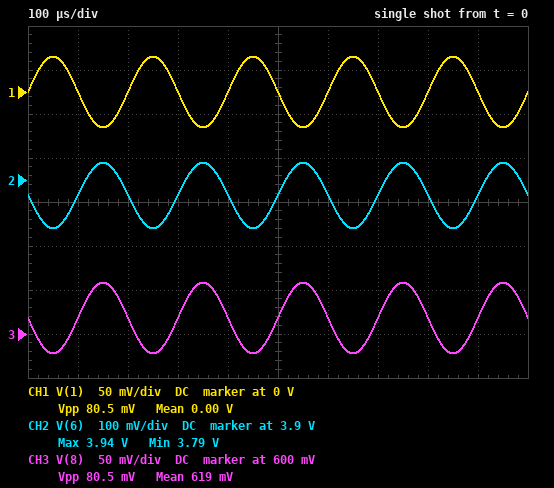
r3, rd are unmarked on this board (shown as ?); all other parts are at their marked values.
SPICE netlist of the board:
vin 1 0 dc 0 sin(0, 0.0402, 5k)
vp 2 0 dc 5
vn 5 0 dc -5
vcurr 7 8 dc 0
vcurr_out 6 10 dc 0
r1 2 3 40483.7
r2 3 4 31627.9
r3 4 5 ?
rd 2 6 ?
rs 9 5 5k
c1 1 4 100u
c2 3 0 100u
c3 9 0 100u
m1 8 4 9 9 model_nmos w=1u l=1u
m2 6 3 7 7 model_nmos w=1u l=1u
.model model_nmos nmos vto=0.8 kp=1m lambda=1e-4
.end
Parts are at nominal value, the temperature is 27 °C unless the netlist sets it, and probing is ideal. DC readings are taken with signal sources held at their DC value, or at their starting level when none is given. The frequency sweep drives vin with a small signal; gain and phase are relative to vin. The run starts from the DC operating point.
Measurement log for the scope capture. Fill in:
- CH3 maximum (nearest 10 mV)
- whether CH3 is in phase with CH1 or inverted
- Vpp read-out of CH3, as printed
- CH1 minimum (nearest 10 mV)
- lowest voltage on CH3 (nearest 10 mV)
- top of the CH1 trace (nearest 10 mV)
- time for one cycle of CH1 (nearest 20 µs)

660 mV
inverted
80.5 mV
-40 mV
580 mV
40 mV
200 µs
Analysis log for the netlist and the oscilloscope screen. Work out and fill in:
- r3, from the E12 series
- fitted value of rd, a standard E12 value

100 kΩ
1.5 kΩ
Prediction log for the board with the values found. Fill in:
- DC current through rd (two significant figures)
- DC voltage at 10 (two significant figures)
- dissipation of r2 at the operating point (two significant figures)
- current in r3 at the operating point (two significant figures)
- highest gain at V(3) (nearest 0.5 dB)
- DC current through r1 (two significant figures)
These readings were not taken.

760 µA
3.9 V
110 µW
58 µA
-10.0 dB
58 µA
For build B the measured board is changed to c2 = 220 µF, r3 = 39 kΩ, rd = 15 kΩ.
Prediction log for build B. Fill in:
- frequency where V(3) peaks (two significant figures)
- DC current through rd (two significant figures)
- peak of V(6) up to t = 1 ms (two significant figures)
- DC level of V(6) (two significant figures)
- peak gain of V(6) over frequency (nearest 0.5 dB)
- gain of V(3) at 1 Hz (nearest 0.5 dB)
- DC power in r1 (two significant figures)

51 mHz
370 µA
-43 mV
-550 mV
22.0 dB
-33.0 dB
330 µW
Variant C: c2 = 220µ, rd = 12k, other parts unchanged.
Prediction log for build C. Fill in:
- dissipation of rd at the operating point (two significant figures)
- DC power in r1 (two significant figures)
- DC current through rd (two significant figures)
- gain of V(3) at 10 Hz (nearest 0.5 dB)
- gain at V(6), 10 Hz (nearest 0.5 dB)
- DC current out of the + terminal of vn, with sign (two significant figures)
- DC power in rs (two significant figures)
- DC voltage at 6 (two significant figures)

3.8 mW
140 µW
560 µA
-53.0 dB
-17.0 dB
-620 µA
1.6 mW
-1.8 V
